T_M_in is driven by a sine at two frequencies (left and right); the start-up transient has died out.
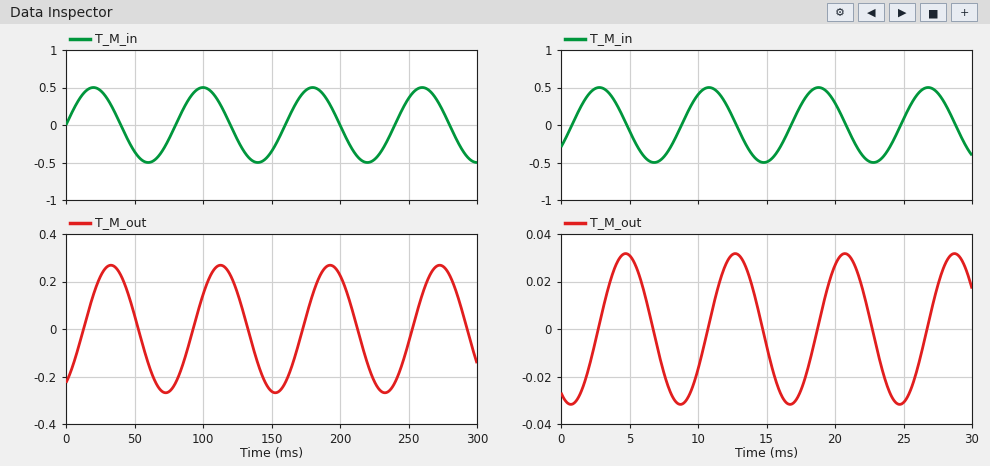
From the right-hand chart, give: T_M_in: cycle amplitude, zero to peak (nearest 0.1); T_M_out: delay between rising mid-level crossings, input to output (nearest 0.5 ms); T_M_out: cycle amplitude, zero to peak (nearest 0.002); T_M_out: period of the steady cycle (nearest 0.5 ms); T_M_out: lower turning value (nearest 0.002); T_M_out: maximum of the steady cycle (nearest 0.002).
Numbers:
0.5
2.0 ms
0.032
8.0 ms
-0.032
0.032
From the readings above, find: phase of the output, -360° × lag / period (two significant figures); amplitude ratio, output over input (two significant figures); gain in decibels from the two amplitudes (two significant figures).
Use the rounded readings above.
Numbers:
-90°
0.064
-24 dB
